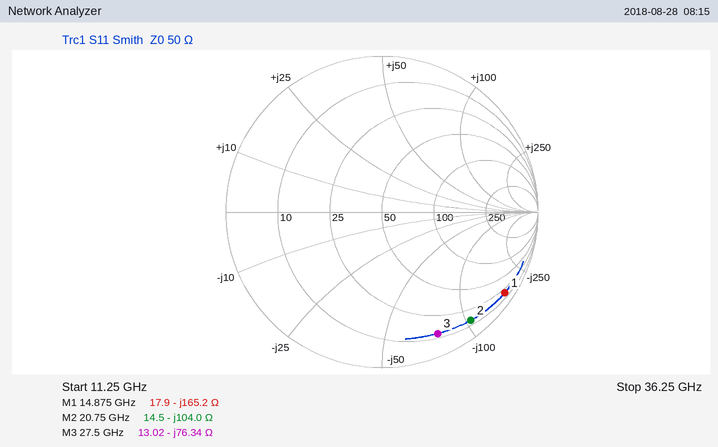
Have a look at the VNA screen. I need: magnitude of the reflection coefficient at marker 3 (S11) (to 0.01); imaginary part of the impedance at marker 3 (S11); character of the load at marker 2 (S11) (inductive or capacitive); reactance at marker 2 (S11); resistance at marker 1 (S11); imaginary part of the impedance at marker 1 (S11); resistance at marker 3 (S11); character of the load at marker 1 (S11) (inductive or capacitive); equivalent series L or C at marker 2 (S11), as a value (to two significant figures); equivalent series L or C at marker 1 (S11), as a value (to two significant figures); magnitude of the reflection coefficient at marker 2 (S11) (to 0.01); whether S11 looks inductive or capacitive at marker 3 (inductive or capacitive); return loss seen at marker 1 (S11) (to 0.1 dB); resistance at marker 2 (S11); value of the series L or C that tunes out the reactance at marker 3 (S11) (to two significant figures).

0.86
-76.34 Ω
capacitive
-104.0 Ω
17.9 Ω
-165.2 Ω
13.02 Ω
capacitive
74 fF
65 fF
0.90
capacitive
0.5 dB
14.5 Ω
440 pH
